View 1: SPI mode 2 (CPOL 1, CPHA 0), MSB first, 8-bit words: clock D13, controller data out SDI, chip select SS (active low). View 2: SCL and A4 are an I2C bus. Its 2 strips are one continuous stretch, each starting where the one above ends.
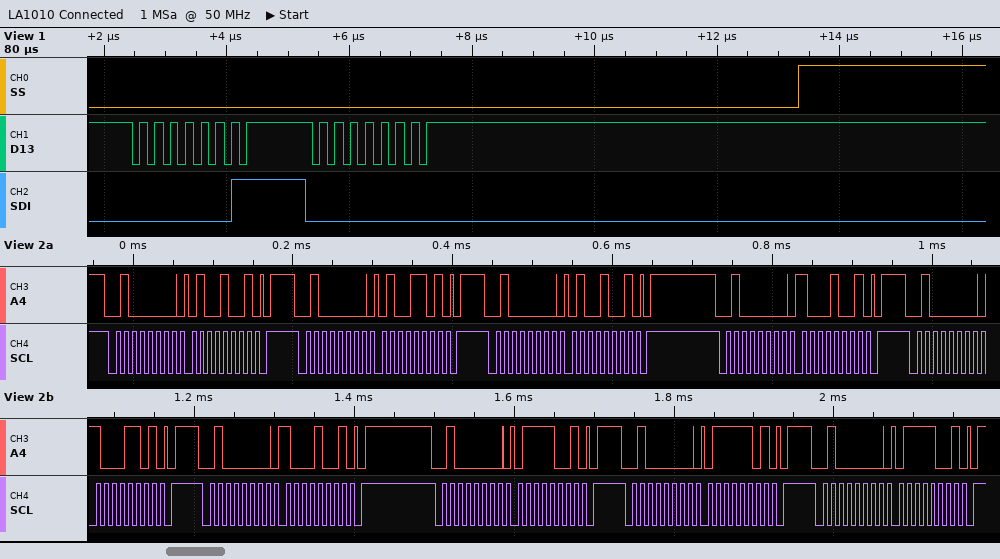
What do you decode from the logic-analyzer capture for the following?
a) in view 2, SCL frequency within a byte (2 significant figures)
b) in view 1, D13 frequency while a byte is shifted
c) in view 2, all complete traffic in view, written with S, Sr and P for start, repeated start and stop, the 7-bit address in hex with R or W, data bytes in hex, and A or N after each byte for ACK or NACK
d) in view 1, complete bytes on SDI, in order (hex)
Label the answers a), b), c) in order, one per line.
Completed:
a) 100 kHz
b) 4 MHz
c) S 20W A 49 A P S 20W A 4D A P S 20W A 49 A P S 20W A 89 A P S 20W A 8D A P S 20W A 89 A P S 20W A 79 A P S 20W A 7D A P S 20W A 79 A P
d) 01 00
